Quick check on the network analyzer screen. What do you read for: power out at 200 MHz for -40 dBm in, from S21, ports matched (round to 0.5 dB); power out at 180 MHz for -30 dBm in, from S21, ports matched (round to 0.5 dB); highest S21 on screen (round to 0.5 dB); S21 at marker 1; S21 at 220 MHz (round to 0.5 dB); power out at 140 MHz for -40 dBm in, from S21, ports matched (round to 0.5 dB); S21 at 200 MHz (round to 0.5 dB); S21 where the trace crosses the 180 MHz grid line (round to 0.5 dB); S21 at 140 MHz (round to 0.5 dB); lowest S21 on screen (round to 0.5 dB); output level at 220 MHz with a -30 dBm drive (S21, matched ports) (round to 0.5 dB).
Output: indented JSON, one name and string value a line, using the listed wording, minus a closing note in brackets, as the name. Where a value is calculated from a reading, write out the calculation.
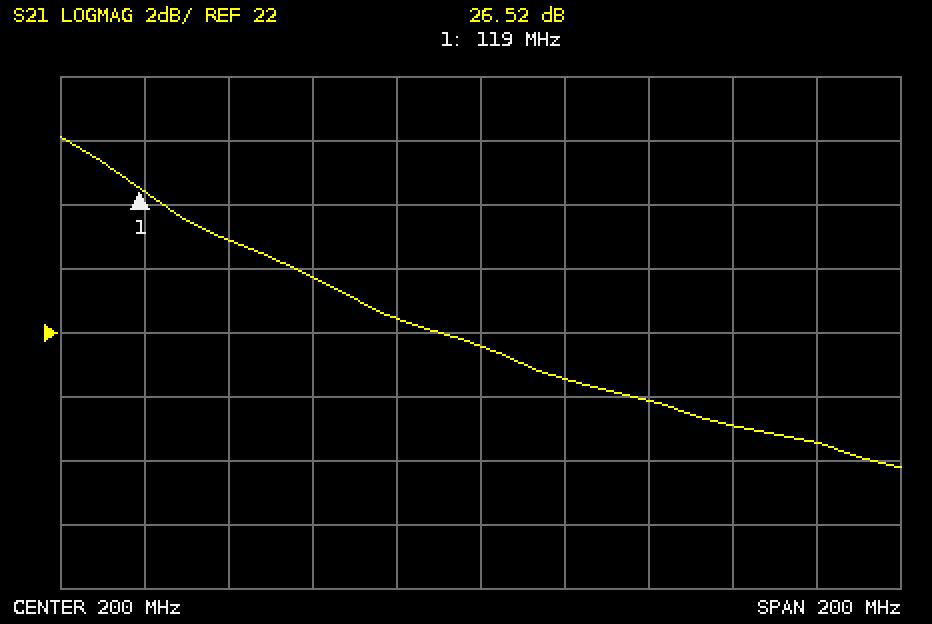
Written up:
{
  "power out at 200 MHz for -40 dBm in, from S21, ports matched": "-40 dBm + (21.5 dB) = -18.5 dBm",
  "power out at 180 MHz for -30 dBm in, from S21, ports matched": "-30 dBm + (22.5 dB) = -7.5 dBm",
  "highest S21 on screen": "28.0 dB",
  "S21 at marker 1": "26.52 dB",
  "S21 at 220 MHz": "20.5 dB",
  "power out at 140 MHz for -40 dBm in, from S21, ports matched": "-40 dBm + (25.0 dB) = -15.0 dBm",
  "S21 at 200 MHz": "21.5 dB",
  "S21 where the trace crosses the 180 MHz grid line": "22.5 dB",
  "S21 at 140 MHz": "25.0 dB",
  "lowest S21 on screen": "18.0 dB",
  "output level at 220 MHz with a -30 dBm drive (S21, matched ports)": "-30 dBm + (20.5 dB) = -9.5 dBm"
}
